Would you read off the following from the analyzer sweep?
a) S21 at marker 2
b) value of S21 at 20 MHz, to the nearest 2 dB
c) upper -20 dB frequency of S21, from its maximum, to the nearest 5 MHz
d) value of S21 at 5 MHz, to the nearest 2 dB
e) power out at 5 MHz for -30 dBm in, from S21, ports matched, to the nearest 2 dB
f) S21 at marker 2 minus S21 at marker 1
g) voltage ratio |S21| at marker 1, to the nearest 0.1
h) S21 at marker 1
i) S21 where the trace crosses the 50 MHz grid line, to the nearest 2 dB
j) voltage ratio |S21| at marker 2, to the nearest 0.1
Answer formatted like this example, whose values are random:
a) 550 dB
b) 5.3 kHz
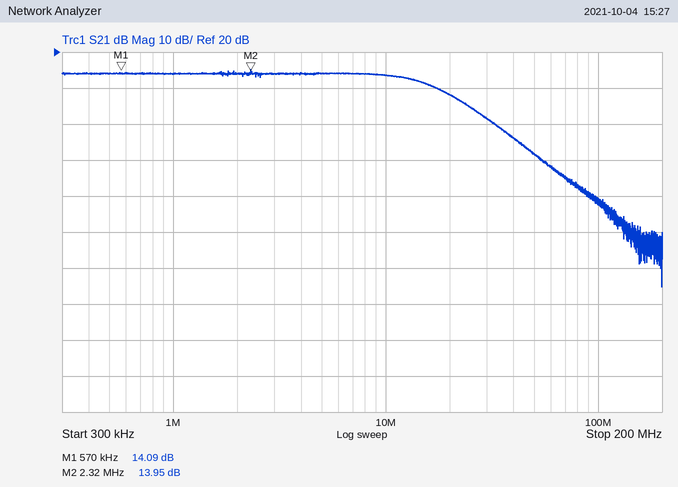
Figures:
a) 13.95 dB
b) 8 dB
c) 40 MHz
d) 14 dB
e) -16 dBm
f) -0.14 dB
g) 5.1
h) 14.09 dB
i) -8 dB
j) 5.0
